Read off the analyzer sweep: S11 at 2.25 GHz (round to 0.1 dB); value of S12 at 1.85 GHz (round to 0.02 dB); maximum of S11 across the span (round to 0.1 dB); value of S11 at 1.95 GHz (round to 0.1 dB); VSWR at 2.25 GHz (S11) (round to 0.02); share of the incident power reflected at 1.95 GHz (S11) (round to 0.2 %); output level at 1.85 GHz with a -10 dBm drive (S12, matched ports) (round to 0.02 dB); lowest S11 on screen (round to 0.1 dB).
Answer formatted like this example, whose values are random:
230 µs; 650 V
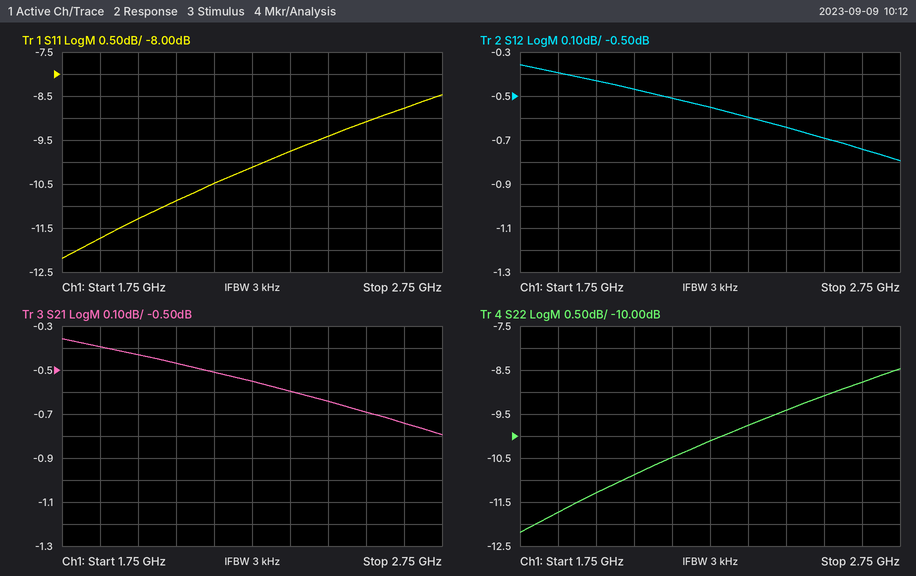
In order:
-10.1 dB; -0.40 dB; -8.5 dB; -11.3 dB; 1.90; 7.4 %; -10.40 dBm; -12.2 dB
